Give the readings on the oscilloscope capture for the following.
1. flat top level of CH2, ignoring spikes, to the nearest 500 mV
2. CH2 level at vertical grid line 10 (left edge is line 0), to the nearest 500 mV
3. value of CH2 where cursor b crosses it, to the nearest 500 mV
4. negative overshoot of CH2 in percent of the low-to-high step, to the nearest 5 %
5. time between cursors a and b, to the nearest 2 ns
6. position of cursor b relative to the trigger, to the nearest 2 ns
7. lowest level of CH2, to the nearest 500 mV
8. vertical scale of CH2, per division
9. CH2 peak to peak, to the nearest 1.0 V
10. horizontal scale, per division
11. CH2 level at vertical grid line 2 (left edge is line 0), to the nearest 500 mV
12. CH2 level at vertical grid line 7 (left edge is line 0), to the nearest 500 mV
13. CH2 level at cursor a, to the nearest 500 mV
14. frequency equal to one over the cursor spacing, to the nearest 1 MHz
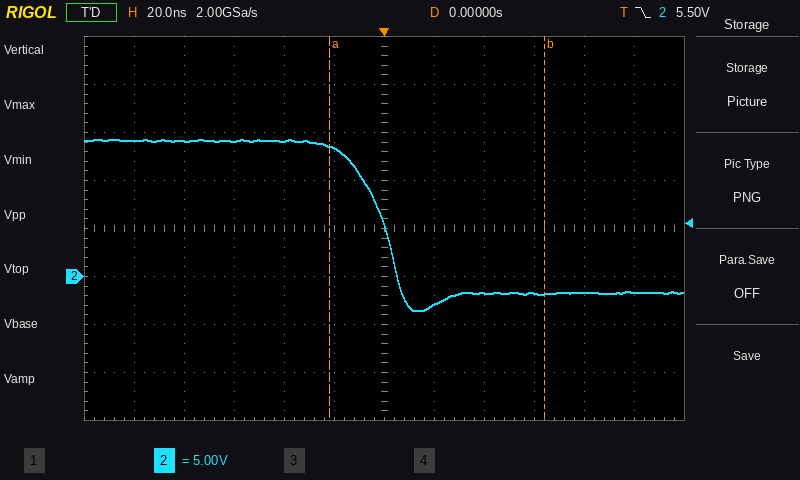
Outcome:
14.0 V
-1.5 V
-2.0 V
10 %
86 ns
+64 ns
-3.5 V
5 V
18.0 V
20 ns
14.0 V
-3.0 V
13.5 V
12 MHz
